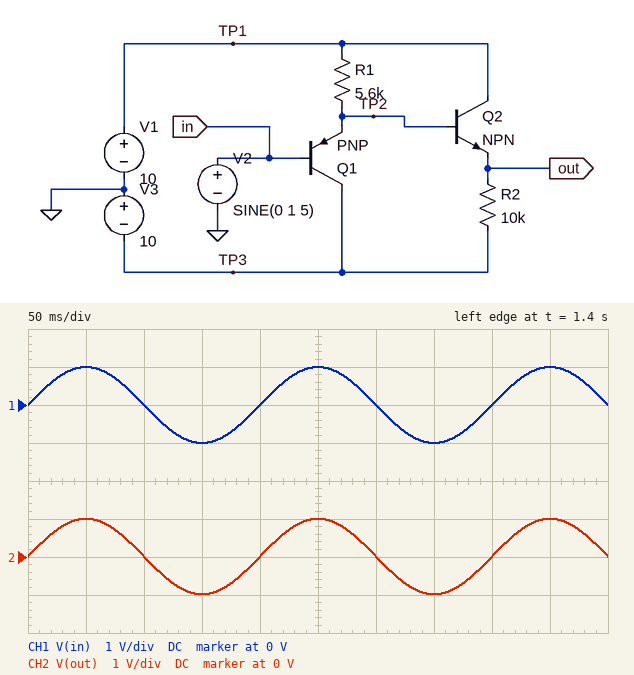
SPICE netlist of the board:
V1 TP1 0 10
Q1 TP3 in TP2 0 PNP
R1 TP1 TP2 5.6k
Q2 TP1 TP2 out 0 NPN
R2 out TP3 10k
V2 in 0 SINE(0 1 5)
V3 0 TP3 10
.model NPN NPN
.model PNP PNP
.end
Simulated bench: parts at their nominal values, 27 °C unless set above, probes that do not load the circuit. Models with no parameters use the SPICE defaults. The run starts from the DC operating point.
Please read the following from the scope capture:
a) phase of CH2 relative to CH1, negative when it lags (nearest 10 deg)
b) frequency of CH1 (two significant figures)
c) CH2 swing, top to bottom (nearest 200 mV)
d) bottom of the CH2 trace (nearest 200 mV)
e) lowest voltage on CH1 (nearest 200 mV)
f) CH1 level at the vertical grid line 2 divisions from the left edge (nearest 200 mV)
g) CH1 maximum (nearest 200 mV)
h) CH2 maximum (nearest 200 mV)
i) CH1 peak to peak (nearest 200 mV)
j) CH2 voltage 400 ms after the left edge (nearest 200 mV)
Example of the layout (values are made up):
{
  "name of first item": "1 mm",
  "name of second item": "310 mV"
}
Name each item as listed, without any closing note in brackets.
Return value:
{
  "phase of CH2 relative to CH1, negative when it lags": "0 deg",
  "frequency of CH1": "5.0 Hz",
  "CH2 swing, top to bottom": "2.0 V",
  "bottom of the CH2 trace": "-1.0 V",
  "lowest voltage on CH1": "-1.0 V",
  "CH1 level at the vertical grid line 2 divisions from the left edge": "0 V",
  "CH1 maximum": "1.0 V",
  "CH2 maximum": "1.0 V",
  "CH1 peak to peak": "2.0 V",
  "CH2 voltage 400 ms after the left edge": "0 V"
}
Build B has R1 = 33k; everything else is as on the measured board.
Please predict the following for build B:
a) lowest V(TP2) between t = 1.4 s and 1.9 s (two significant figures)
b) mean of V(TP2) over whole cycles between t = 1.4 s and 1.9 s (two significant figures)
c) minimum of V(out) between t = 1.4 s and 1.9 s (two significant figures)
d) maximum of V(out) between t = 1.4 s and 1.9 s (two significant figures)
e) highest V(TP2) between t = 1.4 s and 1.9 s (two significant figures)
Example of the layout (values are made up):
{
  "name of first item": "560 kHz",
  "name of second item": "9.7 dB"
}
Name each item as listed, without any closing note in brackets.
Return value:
{
  "lowest V(TP2) between t = 1.4 s and 1.9 s": "-260 mV",
  "mean of V(TP2) over whole cycles between t = 1.4 s and 1.9 s": "740 mV",
  "minimum of V(out) between t = 1.4 s and 1.9 s": "-1.0 V",
  "maximum of V(out) between t = 1.4 s and 1.9 s": "960 mV",
  "highest V(TP2) between t = 1.4 s and 1.9 s": "1.7 V"
}
